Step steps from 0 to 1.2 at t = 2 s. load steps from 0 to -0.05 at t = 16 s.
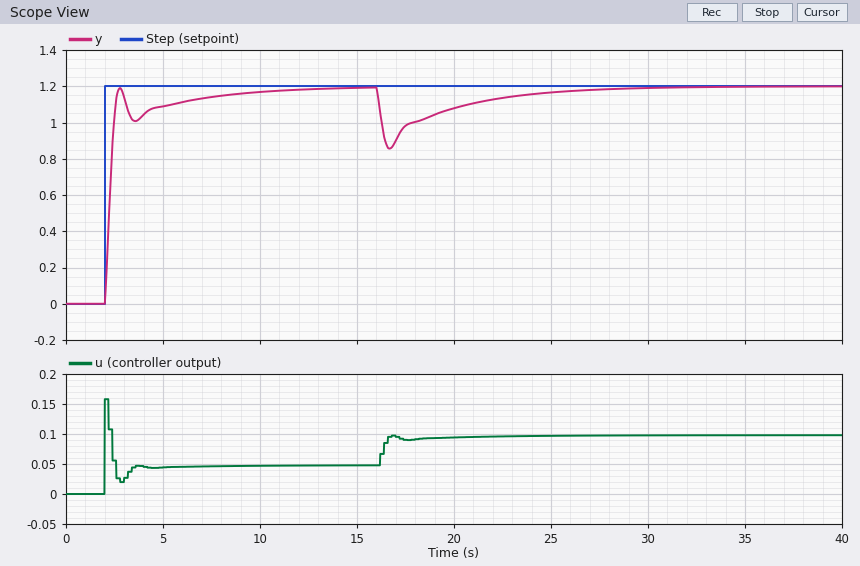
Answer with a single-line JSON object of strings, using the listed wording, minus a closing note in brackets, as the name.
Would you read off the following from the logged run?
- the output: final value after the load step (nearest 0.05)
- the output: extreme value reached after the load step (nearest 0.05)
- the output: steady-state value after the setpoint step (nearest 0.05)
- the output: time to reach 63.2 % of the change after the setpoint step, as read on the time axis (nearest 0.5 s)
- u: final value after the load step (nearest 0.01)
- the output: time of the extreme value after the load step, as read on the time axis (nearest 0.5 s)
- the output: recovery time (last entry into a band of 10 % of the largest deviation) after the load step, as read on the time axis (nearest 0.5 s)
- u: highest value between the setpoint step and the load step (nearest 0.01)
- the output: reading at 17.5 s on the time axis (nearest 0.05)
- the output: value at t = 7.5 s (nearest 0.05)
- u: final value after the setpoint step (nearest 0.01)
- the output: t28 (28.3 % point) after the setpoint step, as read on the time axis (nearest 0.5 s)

{"the output: final value after the load step": "1.20", "the output: extreme value reached after the load step": "0.85", "the output: steady-state value after the setpoint step": "1.20", "the output: time to reach 63.2 % of the change after the setpoint step, as read on the time axis": "2.5 s", "u: final value after the load step": "0.10", "the output: time of the extreme value after the load step, as read on the time axis": "16.5 s", "the output: recovery time (last entry into a band of 10 % of the largest deviation) after the load step, as read on the time axis": "25.0 s", "u: highest value between the setpoint step and the load step": "0.16", "the output: reading at 17.5 s on the time axis": "1.00", "the output: value at t = 7.5 s": "1.15", "u: final value after the setpoint step": "0.05", "the output: t28 (28.3 % point) after the setpoint step, as read on the time axis": "2.0 s"}
